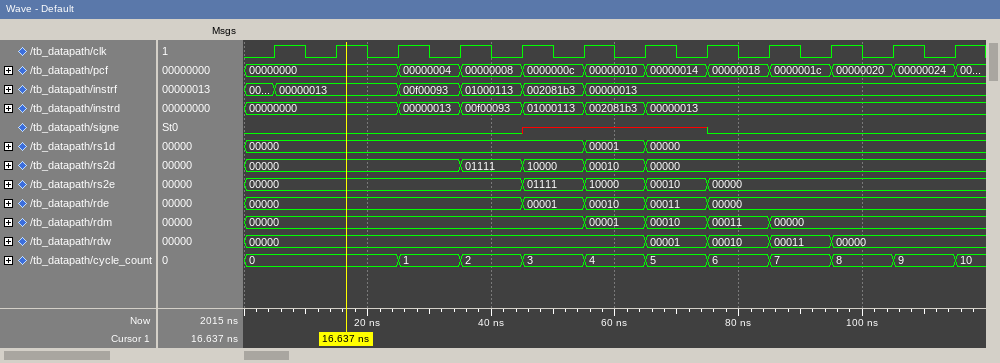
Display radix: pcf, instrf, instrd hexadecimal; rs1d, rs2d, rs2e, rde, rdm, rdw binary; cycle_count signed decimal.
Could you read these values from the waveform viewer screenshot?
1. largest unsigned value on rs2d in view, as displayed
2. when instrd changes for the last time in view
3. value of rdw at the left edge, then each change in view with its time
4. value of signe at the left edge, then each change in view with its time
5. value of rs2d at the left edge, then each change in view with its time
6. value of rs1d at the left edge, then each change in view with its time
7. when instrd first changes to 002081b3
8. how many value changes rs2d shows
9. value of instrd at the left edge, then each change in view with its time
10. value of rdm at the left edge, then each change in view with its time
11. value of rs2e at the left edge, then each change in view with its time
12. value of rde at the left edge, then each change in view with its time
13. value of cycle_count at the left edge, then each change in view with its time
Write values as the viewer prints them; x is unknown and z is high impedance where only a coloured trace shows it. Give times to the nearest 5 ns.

10000
65 ns
00000, 00001 at 65 ns, 00010 at 75 ns, 00011 at 85 ns, 00000 at 95 ns
0, x at 45 ns, 0 at 75 ns
00000, 01111 at 35 ns, 10000 at 45 ns, 00010 at 55 ns, 00000 at 65 ns
00000, 00001 at 55 ns, 00000 at 65 ns
55 ns
4
00000000, 00000013 at 25 ns, 00f00093 at 35 ns, 01000113 at 45 ns, 002081b3 at 55 ns, 00000013 at 65 ns
00000, 00001 at 55 ns, 00010 at 65 ns, 00011 at 75 ns, 00000 at 85 ns
00000, 01111 at 45 ns, 10000 at 55 ns, 00010 at 65 ns, 00000 at 75 ns
00000, 00001 at 45 ns, 00010 at 55 ns, 00011 at 65 ns, 00000 at 75 ns
0, 1 at 25 ns, 2 at 35 ns, 3 at 45 ns, 4 at 55 ns, 5 at 65 ns, 6 at 75 ns, 7 at 85 ns, 8 at 95 ns, 9 at 105 ns, 10 at 115 ns
